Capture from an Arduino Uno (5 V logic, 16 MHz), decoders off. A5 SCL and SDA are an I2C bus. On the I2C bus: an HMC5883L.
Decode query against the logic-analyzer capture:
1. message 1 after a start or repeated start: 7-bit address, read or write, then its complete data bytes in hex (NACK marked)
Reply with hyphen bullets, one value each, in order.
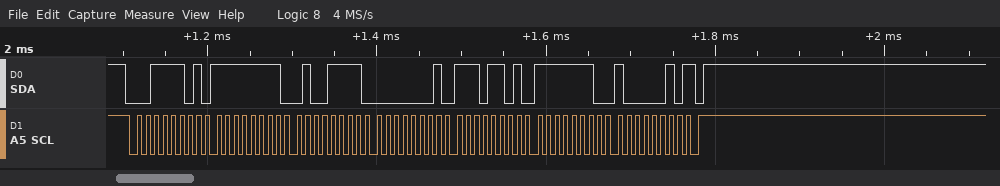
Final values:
- 0x1E read: FF 4F 01 ED FE 82 NACK
